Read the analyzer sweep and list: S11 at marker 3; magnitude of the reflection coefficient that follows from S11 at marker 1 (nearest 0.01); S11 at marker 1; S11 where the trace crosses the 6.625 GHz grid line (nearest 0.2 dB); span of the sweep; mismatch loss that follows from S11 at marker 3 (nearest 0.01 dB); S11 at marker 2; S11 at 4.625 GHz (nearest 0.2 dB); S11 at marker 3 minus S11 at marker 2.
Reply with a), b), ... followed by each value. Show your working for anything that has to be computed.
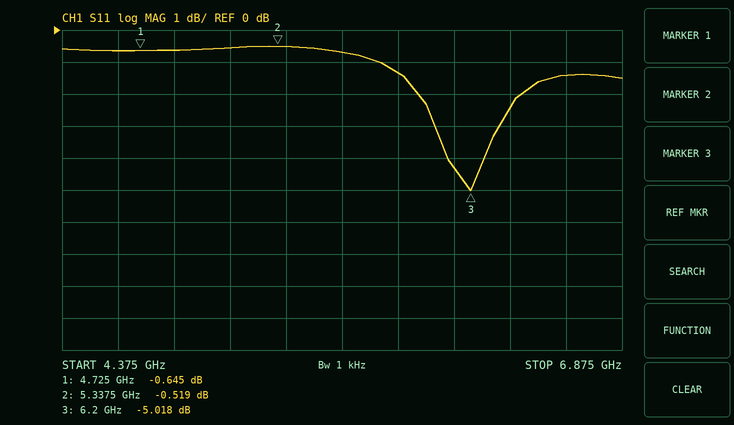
a) -5.018 dB
b) 10^(-0.645/20) ≈ 0.93
c) -0.645 dB
d) -1.4 dB
e) 2.5 GHz
f) −10 log10(1 − 10^(-5.018/10)) ≈ 1.64 dB
g) -0.519 dB
h) -0.6 dB
i) -5.018 − (-0.519) = -4.499 dB
